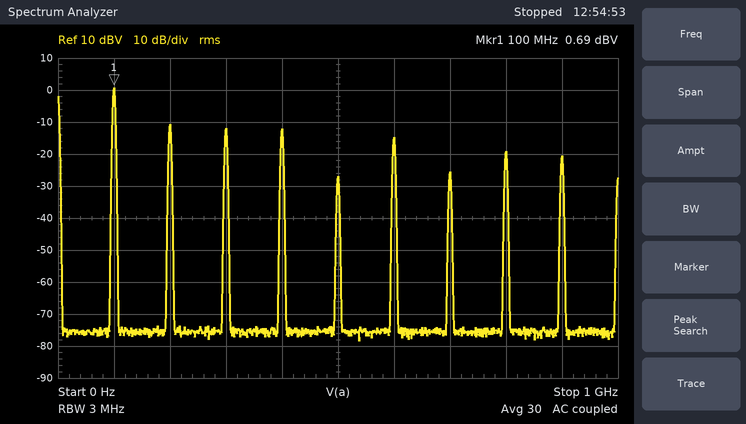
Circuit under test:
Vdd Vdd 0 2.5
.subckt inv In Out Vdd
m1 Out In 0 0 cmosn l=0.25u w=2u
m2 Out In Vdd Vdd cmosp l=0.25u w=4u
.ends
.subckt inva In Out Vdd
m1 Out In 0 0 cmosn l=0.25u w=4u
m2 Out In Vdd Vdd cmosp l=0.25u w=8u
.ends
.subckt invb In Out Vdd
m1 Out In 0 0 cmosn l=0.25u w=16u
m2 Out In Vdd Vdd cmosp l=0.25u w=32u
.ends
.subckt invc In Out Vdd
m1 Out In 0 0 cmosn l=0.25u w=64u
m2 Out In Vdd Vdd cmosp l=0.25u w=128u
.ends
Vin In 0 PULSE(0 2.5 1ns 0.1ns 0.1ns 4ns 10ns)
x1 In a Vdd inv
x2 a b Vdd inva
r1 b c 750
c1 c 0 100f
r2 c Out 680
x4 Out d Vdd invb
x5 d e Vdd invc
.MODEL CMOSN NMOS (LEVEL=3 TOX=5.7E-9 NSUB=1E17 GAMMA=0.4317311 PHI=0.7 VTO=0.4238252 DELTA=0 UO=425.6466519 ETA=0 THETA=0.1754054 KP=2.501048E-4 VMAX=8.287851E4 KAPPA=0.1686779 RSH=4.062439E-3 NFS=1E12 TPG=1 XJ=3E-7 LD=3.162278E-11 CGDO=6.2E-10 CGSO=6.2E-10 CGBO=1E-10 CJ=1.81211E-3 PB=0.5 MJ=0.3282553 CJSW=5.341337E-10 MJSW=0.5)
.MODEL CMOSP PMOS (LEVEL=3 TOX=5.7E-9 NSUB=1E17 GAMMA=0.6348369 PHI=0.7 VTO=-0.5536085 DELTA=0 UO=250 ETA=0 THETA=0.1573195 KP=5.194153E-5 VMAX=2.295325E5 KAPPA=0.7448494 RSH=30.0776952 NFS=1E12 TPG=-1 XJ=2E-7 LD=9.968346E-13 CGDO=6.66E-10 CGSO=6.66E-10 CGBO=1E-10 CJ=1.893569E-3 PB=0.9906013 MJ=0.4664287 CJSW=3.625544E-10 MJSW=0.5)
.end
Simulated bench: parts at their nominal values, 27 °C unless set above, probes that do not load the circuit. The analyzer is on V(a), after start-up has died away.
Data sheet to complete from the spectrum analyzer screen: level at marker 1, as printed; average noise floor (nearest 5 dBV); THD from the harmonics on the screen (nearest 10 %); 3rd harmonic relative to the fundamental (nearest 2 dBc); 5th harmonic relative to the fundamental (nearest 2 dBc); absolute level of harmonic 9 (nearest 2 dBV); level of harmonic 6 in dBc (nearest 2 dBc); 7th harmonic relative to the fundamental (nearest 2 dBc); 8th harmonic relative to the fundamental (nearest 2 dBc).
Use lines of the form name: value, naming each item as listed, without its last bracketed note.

level at marker 1, as printed: 0.69 dBV
average noise floor: -75 dBV
THD from the harmonics on the screen: 50 %
3rd harmonic relative to the fundamental: -12 dBc
5th harmonic relative to the fundamental: -28 dBc
absolute level of harmonic 9: -20 dBV
level of harmonic 6 in dBc: -16 dBc
7th harmonic relative to the fundamental: -26 dBc
8th harmonic relative to the fundamental: -20 dBc
